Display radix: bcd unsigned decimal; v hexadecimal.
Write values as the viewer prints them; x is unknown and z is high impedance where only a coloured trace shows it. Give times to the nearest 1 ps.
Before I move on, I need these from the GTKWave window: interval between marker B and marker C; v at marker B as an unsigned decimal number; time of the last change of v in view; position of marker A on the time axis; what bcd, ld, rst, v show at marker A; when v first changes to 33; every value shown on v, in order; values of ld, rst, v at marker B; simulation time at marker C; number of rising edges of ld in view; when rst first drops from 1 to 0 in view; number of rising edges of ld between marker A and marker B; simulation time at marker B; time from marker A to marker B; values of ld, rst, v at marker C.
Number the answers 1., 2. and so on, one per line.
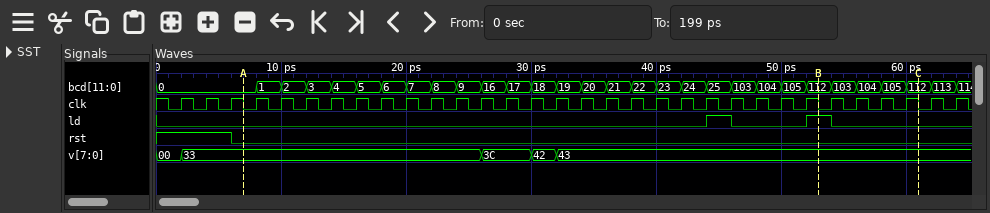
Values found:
1. 8 ps
2. 67
3. 32 ps
4. 7 ps
5. bcd=0, ld=0, rst=0, v=33
6. 2 ps
7. 00, 33, 3C, 42, 43
8. ld=1, rst=0, v=43
9. 61 ps
10. 2
11. 6 ps
12. 2
13. 53 ps
14. 46 ps
15. ld=0, rst=0, v=43
